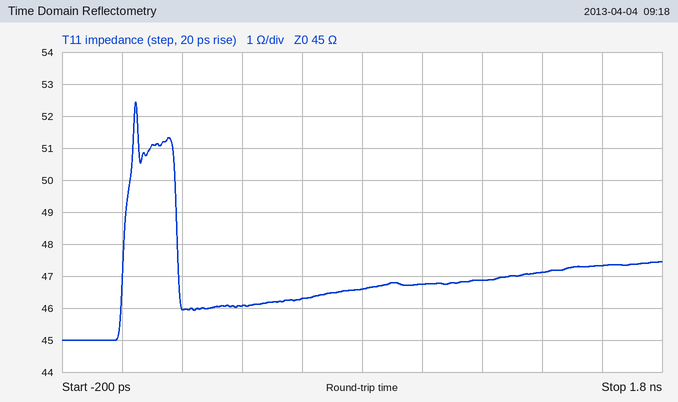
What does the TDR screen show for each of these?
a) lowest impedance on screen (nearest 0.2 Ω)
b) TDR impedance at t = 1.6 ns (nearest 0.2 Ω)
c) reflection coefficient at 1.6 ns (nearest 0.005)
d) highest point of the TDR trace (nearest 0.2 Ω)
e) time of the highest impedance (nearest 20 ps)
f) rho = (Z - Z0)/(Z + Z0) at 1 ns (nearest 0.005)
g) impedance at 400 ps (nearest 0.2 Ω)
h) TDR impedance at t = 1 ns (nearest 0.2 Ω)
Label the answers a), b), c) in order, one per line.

a) 45.0 Ω
b) 47.4 Ω
c) +0.025
d) 52.4 Ω
e) 40 ps
f) +0.020
g) 46.0 Ω
h) 46.8 Ω
